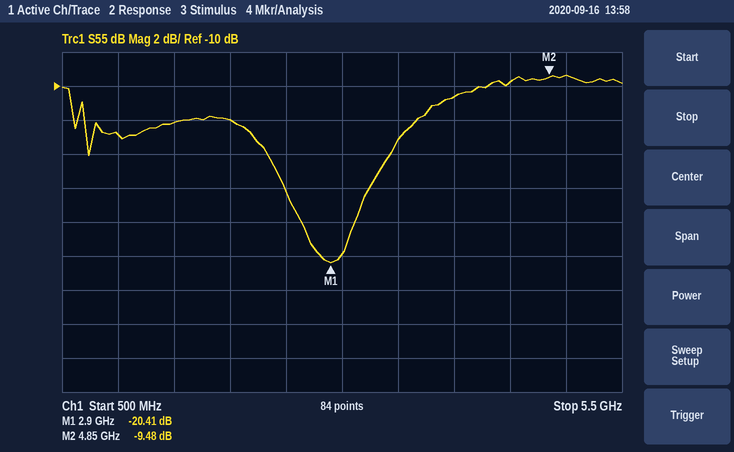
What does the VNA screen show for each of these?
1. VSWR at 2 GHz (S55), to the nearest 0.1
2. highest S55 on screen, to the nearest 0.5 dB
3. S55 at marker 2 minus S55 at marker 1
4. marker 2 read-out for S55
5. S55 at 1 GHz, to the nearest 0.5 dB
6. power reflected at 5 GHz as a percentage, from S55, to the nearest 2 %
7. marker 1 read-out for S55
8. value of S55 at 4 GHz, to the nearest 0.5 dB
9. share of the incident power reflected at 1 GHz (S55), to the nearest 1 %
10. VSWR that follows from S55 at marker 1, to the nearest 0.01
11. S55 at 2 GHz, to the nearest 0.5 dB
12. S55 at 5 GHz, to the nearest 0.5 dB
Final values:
1.7
-9.5 dB
10.93 dB
-9.48 dB
-13.0 dB
12 %
-20.41 dB
-10.5 dB
5 %
1.21
-12.0 dB
-9.5 dB
